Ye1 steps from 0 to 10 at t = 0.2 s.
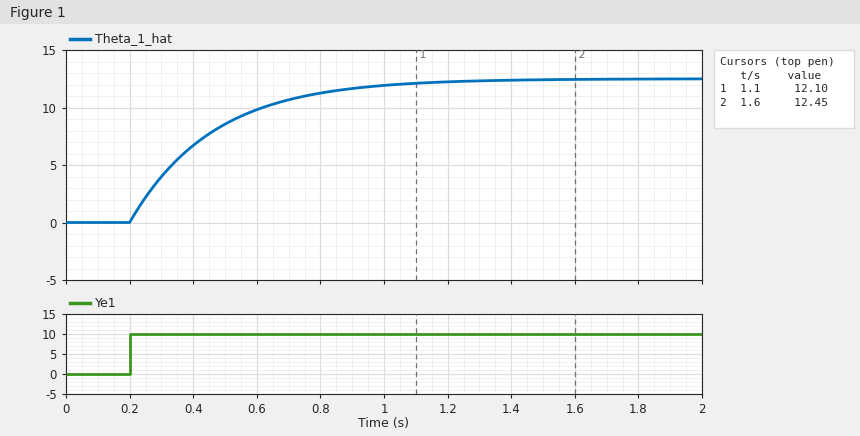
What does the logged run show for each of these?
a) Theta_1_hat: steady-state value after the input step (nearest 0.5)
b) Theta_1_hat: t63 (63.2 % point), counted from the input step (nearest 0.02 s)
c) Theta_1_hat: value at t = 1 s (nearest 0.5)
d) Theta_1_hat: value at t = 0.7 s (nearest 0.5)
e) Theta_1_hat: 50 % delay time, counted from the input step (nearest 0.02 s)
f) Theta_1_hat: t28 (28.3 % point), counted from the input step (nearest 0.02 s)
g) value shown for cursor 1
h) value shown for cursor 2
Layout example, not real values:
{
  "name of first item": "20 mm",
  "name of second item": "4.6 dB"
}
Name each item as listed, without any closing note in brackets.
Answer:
{
  "Theta_1_hat: steady-state value after the input step": "12.5",
  "Theta_1_hat: t63 (63.2 % point), counted from the input step": "0.26 s",
  "Theta_1_hat: value at t = 1 s": "12.0",
  "Theta_1_hat: value at t = 0.7 s": "10.5",
  "Theta_1_hat: 50 % delay time, counted from the input step": "0.18 s",
  "Theta_1_hat: t28 (28.3 % point), counted from the input step": "0.08 s",
  "value shown for cursor 1": "12.10",
  "value shown for cursor 2": "12.45"
}
